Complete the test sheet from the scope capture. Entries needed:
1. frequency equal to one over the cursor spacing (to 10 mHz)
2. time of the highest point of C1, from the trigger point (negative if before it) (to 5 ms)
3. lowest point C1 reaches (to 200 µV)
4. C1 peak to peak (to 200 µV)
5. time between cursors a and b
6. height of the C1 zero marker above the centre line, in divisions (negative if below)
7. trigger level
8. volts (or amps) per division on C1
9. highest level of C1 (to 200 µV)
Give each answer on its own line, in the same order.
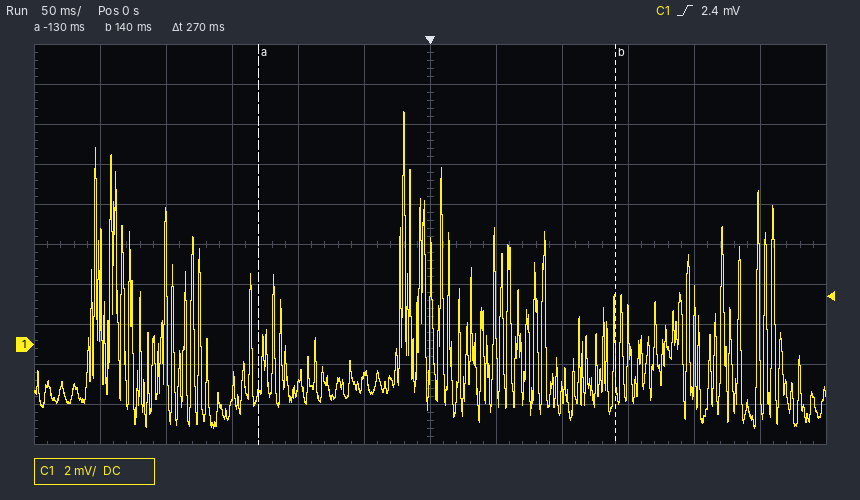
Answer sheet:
3.70 Hz
-20 ms
-4.2 mV
15.8 mV
270 ms
-2.5 div
2.4 mV
2 mV
11.6 mV
